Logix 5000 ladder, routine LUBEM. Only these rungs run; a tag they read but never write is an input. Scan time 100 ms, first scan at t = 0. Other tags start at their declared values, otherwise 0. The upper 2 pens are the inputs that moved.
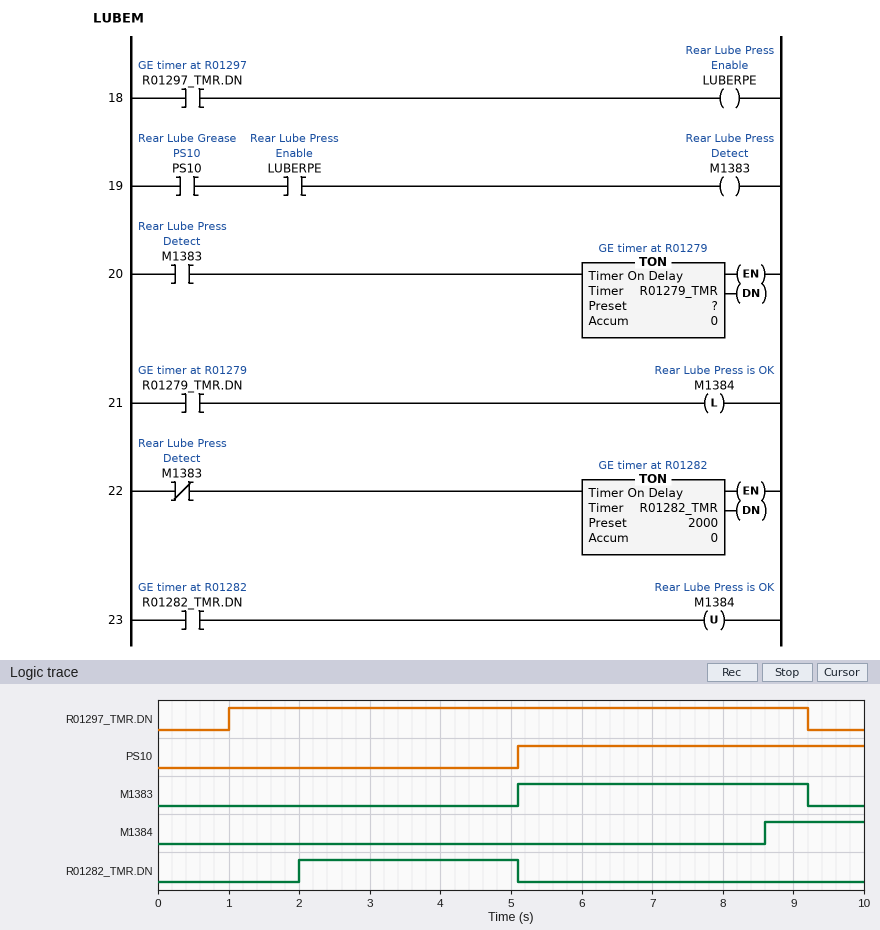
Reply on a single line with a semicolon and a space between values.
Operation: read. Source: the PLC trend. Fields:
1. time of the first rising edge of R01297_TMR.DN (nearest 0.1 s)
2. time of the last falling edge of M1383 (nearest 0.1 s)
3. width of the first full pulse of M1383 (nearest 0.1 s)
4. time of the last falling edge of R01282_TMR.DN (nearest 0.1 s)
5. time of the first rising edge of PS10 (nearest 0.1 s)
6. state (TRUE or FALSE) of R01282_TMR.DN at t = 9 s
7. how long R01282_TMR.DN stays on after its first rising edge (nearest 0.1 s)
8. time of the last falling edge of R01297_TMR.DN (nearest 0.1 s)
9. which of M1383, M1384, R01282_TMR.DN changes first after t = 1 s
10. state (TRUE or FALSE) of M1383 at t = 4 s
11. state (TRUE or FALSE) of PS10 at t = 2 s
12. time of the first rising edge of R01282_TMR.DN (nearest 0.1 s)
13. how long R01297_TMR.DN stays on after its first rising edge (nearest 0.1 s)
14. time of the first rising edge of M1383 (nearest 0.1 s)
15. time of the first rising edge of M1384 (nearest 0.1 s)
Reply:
1.0 s; 9.2 s; 4.1 s; 5.1 s; 5.1 s; FALSE; 3.1 s; 9.2 s; R01282_TMR.DN; FALSE; FALSE; 2.0 s; 8.2 s; 5.1 s; 8.6 s
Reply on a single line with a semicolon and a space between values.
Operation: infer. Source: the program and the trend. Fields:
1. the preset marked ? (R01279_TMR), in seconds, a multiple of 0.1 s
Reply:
3.5 s
